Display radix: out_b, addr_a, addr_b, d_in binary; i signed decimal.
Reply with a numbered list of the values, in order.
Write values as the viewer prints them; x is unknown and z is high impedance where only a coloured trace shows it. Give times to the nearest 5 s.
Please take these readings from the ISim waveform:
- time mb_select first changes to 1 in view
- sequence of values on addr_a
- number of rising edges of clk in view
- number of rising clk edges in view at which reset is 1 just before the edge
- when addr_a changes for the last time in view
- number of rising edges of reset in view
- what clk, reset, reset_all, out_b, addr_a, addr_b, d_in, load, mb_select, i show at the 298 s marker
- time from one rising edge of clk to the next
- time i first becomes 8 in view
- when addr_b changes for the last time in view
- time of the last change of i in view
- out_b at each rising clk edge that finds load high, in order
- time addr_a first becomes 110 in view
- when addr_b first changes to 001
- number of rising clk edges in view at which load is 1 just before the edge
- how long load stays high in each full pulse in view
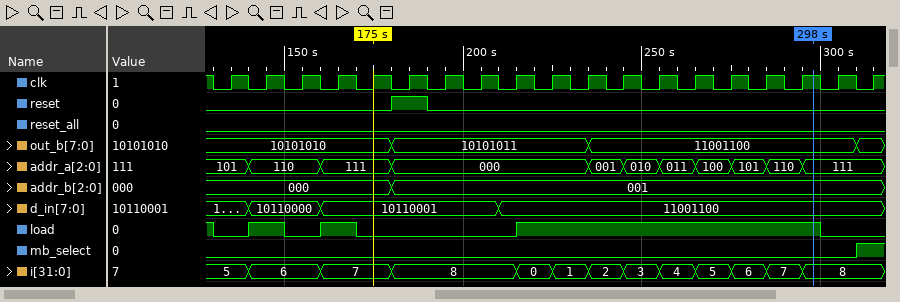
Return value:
1. 310 s
2. 101, 110, 111, 000, 001, 010, 011, 100, 101, 110, 111
3. 19
4. 1
5. 295 s
6. 1
7. clk=1, reset=0, reset_all=0, out_b=11001100, addr_a=111, addr_b=001, d_in=11001100, load=1, mb_select=0, i=8
8. 10 s
9. 180 s
10. 180 s
11. 295 s
12. 10101010, 10101010, 10101011, 10101011, 11001100, 11001100, 11001100, 11001100, 11001100, 11001100
13. 140 s
14. 180 s
15. 10
16. 10 s, 10 s, 85 s
